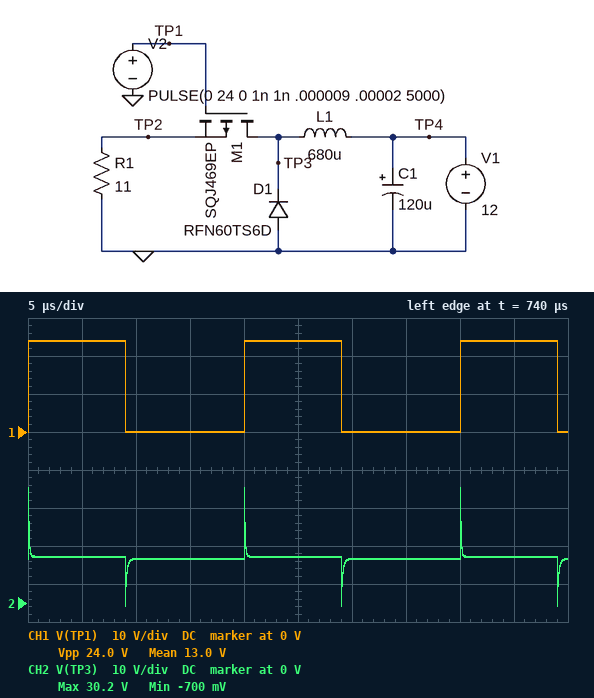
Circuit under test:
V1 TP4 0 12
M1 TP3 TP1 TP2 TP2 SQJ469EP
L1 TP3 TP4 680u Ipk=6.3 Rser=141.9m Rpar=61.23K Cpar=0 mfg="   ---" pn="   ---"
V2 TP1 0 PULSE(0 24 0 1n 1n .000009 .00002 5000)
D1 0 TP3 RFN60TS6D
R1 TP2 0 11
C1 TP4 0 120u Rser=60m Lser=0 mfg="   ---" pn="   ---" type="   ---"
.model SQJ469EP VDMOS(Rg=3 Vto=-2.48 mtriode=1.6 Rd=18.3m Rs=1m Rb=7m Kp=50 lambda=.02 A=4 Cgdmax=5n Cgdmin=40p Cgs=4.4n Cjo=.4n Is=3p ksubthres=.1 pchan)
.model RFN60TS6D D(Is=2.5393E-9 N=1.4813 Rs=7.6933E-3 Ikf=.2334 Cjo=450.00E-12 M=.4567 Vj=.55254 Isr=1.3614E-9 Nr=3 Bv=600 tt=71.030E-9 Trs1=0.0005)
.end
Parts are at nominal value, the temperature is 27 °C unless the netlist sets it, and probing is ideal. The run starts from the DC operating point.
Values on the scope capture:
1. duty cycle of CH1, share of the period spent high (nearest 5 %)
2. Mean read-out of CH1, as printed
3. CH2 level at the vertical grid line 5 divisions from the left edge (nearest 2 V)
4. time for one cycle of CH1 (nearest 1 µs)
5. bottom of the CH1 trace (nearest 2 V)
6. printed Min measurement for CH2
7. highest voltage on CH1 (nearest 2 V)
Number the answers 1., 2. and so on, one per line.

1. 45 %
2. 13.0 V
3. 12 V
4. 20 µs
5. 0 V
6. -700 mV
7. 24 V
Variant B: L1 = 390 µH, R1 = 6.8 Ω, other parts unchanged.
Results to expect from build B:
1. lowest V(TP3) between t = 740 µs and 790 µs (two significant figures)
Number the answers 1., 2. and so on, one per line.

1. -680 mV
